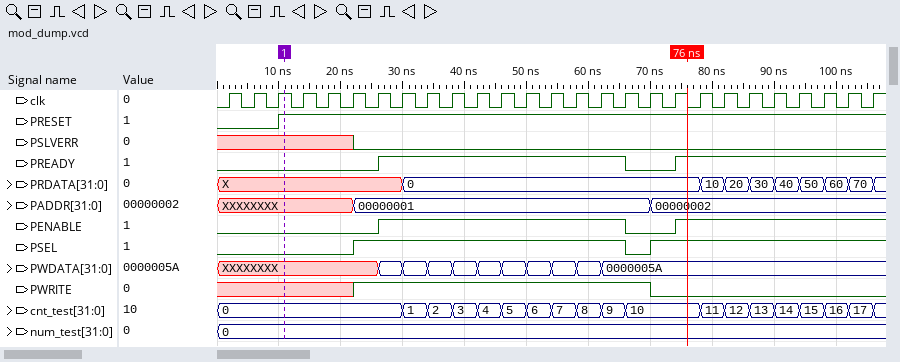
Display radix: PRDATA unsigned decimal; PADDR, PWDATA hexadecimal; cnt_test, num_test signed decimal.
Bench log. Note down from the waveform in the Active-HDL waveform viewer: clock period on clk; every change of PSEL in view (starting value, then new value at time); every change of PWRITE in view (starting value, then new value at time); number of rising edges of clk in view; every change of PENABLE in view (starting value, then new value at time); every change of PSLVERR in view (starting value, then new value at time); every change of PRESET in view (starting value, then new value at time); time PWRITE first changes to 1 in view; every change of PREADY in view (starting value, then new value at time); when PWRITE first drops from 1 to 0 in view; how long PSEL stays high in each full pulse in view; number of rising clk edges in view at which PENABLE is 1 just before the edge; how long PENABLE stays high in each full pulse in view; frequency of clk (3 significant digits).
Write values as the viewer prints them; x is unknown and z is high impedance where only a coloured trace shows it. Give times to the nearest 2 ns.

4 ns
0, 1 at 22 ns, 0 at 66 ns, 1 at 70 ns
x, 1 at 22 ns, 0 at 70 ns
27
0, 1 at 26 ns, 0 at 66 ns, 1 at 74 ns
x, 0 at 22 ns
0, 1 at 10 ns
22 ns
0, 1 at 26 ns, 0 at 66 ns, 1 at 74 ns
70 ns
44 ns
18
40 ns
250 MHz
